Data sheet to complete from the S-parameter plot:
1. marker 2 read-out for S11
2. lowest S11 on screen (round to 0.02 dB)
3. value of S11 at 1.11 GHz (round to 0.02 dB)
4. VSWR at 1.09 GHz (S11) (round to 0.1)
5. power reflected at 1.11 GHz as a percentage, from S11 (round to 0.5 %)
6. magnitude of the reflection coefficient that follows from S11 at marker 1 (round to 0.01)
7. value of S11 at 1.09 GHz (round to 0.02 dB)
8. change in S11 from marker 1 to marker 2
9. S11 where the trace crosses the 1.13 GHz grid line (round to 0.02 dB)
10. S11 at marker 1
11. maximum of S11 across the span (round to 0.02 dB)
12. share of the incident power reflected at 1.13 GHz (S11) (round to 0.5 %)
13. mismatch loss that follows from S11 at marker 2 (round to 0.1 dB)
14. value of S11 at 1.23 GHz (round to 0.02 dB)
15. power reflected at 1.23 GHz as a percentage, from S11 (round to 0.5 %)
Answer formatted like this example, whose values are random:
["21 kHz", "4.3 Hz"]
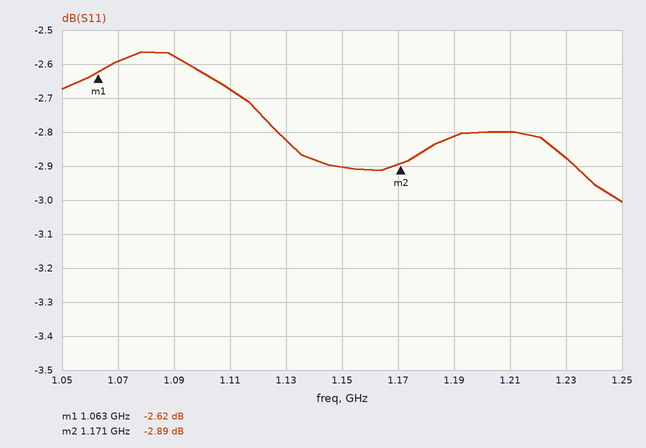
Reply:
["-2.89 dB", "-3.00 dB", "-2.68 dB", "6.8", "54.0 %", "0.74", "-2.58 dB", "-0.27 dB", "-2.82 dB", "-2.62 dB", "-2.56 dB", "52.0 %", "3.1 dB", "-2.88 dB", "51.5 %"]
